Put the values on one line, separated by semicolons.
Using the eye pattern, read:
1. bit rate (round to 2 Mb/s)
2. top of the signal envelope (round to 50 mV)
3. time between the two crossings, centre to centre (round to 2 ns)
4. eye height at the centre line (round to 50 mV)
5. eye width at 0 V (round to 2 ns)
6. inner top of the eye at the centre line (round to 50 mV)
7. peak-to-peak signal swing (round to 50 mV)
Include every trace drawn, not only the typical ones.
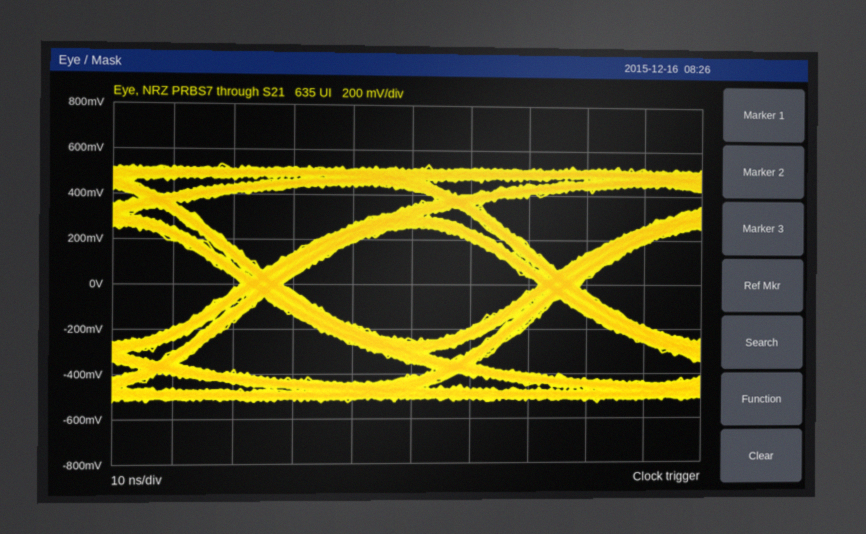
20 Mb/s; 550 mV; 50 ns; 500 mV; 44 ns; 250 mV; 1.05 V
